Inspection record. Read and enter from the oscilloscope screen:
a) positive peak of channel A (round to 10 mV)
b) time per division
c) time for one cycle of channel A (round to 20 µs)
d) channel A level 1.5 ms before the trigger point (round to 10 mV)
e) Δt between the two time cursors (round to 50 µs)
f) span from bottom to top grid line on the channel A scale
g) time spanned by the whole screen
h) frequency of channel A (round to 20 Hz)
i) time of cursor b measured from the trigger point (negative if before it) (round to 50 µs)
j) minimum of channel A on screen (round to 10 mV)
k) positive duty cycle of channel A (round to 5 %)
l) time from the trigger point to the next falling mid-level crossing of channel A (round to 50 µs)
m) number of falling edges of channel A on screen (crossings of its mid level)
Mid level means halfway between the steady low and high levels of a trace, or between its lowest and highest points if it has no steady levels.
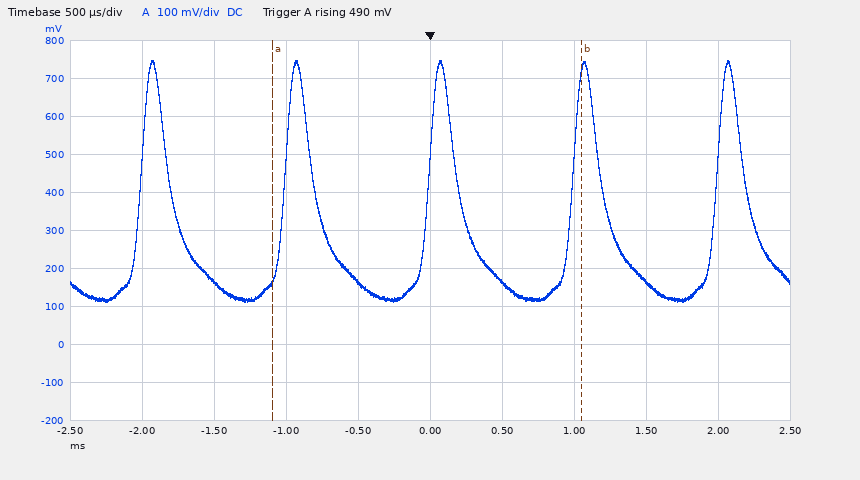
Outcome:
750 mV
500 µs
1.00 ms
170 mV
2.15 ms
1 V
5 ms
1.00 kHz
+1.05 ms
110 mV
20 %
200 µs
5
